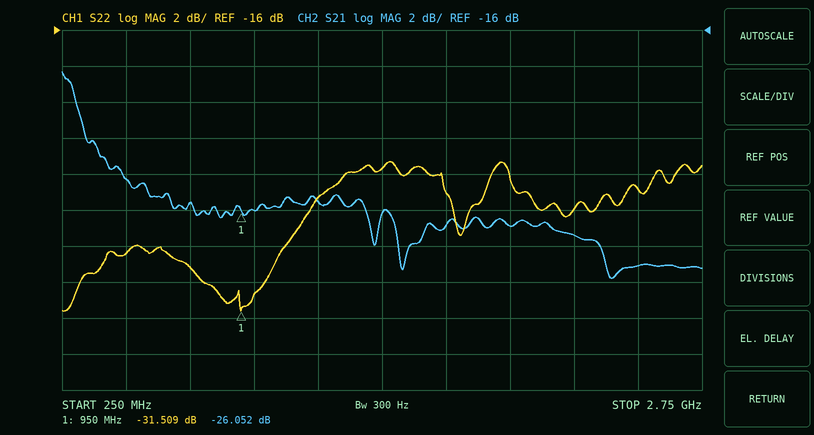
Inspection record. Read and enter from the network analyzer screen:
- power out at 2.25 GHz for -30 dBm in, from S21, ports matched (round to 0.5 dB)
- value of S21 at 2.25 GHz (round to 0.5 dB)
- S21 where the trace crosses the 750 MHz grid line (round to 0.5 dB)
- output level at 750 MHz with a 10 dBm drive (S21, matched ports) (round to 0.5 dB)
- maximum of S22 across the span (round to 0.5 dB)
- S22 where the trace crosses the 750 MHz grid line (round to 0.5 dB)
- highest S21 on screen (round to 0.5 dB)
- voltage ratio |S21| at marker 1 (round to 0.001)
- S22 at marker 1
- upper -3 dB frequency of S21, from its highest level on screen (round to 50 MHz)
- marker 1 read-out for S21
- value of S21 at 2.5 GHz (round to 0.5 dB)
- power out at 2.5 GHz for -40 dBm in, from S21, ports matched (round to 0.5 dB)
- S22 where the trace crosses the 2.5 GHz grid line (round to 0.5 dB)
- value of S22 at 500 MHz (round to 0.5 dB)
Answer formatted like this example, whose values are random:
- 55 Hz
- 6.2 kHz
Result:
- -57.5 dBm
- -27.5 dB
- -25.5 dB
- -15.5 dBm
- -23.5 dB
- -29.0 dB
- -18.5 dB
- 0.050
- -31.509 dB
- 350 MHz
- -26.052 dB
- -29.0 dB
- -69.0 dBm
- -25.0 dB
- -28.5 dB
